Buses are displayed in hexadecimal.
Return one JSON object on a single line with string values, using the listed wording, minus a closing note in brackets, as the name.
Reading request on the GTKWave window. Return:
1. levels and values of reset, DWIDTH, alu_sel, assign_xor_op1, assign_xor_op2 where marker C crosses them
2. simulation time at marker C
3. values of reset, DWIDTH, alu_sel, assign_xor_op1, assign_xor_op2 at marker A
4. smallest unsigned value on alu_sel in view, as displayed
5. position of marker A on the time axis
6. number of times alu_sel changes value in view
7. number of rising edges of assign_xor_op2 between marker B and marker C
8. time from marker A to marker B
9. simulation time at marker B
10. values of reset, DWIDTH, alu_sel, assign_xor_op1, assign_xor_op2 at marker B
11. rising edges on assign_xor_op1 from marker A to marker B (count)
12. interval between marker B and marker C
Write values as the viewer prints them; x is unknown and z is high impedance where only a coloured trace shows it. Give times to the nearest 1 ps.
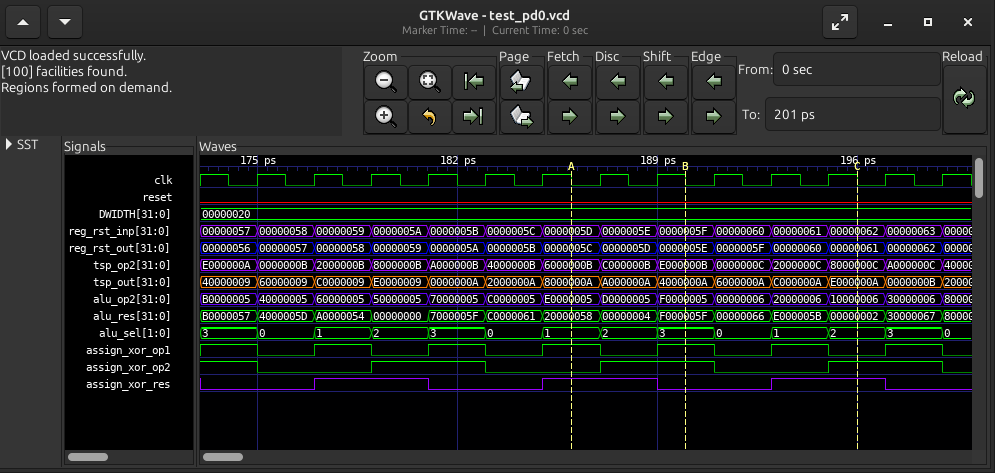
{"levels and values of reset, DWIDTH, alu_sel, assign_xor_op1, assign_xor_op2 where marker C crosses them": "reset=0, DWIDTH=00000020, alu_sel=2, assign_xor_op1=0, assign_xor_op2=1", "simulation time at marker C": "196 ps", "values of reset, DWIDTH, alu_sel, assign_xor_op1, assign_xor_op2 at marker A": "reset=0, DWIDTH=00000020, alu_sel=1, assign_xor_op1=1, assign_xor_op2=0", "smallest unsigned value on alu_sel in view, as displayed": "0", "position of marker A on the time axis": "186 ps", "number of times alu_sel changes value in view": "13", "number of rising edges of assign_xor_op2 between marker B and marker C": "1", "time from marker A to marker B": "4 ps", "simulation time at marker B": "190 ps", "values of reset, DWIDTH, alu_sel, assign_xor_op1, assign_xor_op2 at marker B": "reset=0, DWIDTH=00000020, alu_sel=3, assign_xor_op1=1, assign_xor_op2=1", "rising edges on assign_xor_op1 from marker A to marker B": "1", "interval between marker B and marker C": "6 ps"}
